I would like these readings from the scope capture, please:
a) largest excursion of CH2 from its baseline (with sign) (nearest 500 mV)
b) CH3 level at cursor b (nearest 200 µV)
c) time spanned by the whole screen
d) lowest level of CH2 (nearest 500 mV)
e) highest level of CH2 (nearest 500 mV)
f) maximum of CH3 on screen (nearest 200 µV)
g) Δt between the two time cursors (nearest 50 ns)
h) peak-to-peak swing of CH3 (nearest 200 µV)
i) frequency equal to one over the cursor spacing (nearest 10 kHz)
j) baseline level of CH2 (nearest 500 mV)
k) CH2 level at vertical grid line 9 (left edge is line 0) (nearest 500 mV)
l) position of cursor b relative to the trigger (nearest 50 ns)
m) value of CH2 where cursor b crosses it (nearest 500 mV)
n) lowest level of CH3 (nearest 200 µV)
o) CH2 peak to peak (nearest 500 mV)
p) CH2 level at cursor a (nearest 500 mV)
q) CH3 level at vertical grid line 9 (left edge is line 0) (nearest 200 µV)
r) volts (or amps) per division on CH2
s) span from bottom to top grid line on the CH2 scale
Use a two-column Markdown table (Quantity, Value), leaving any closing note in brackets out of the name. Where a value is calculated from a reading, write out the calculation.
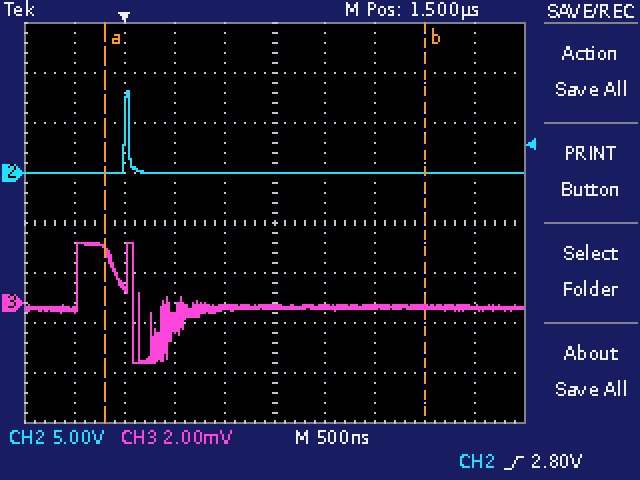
| Quantity | Value |
|---|---|
| largest excursion of CH2 from its baseline (with sign) | 8.0 V − (0.0 V) = +8.0 V |
| CH3 level at cursor b | -200 µV |
| time spanned by the whole screen | 5 µs |
| lowest level of CH2 | 0.0 V |
| highest level of CH2 | 8.0 V |
| maximum of CH3 on screen | 2.4 mV |
| Δt between the two time cursors | 3.20 µs |
| peak-to-peak swing of CH3 | 2.4 mV − (-2.4 mV) = 4.8 mV |
| frequency equal to one over the cursor spacing | 1 / 3.20 µs ≈ 310 kHz |
| baseline level of CH2 | 0.0 V |
| CH2 level at vertical grid line 9 (left edge is line 0) | 0.0 V |
| position of cursor b relative to the trigger | +3.00 µs |
| value of CH2 where cursor b crosses it | 0.0 V |
| lowest level of CH3 | -2.4 mV |
| CH2 peak to peak | 8.0 V − (0.0 V) = 8.0 V |
| CH2 level at cursor a | 0.0 V |
| CH3 level at vertical grid line 9 (left edge is line 0) | -200 µV |
| volts (or amps) per division on CH2 | 5 V |
| span from bottom to top grid line on the CH2 scale | 40 V |
